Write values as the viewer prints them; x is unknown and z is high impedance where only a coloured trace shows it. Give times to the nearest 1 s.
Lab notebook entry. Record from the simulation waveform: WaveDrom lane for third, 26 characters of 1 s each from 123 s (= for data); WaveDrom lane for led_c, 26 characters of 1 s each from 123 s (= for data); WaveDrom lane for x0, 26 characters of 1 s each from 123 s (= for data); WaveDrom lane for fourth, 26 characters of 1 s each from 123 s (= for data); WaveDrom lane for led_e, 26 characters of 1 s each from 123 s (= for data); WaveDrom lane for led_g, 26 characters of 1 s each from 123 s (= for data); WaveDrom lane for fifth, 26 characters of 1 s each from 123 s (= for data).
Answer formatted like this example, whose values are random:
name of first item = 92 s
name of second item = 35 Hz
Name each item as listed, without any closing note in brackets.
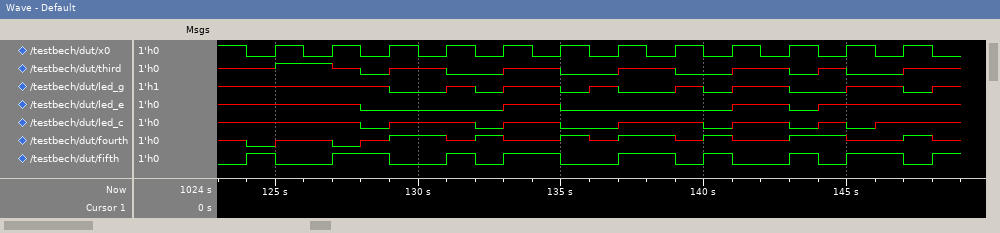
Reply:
WaveDrom lane for third, 26 characters of 1 s each from 123 s = {name: 'third', wave: 'x.1.x0x.0.x.0.x.0.x.0x0.x.'}
WaveDrom lane for led_c, 26 characters of 1 s each from 123 s = {name: 'led_c', wave: 'x....0x..0x.0.x..0x.0x0x..'}
WaveDrom lane for x0, 26 characters of 1 s each from 123 s = {name: 'x0', wave: '10101010101010101010101010'}
WaveDrom lane for fourth, 26 characters of 1 s each from 123 s = {name: 'fourth', wave: 'x0x.0x1.x1x.1x1.x1x.1.x.1x'}
WaveDrom lane for led_e, 26 characters of 1 s each from 123 s = {name: 'led_e', wave: 'x....0....x.0.....x.0x....'}
WaveDrom lane for led_g, 26 characters of 1 s each from 123 s = {name: 'led_g', wave: 'x.....0.x0x.0x0.x0x.0.x.0x'}
WaveDrom lane for fifth, 26 characters of 1 s each from 123 s = {name: 'fifth', wave: '010.1.0.101.0.1.010.101.01'}
